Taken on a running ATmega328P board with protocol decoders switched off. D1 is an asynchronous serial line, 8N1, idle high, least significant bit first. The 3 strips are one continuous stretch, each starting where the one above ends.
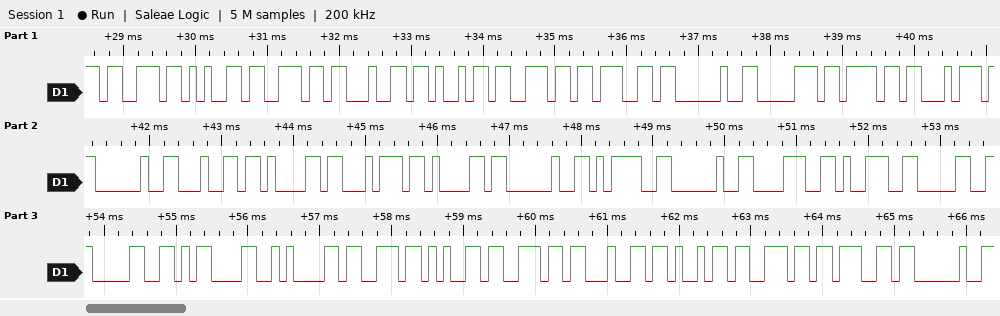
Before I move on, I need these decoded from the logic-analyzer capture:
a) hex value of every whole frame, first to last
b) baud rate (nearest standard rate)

73 65 6E 64 69 6E 67 20 70 6F 74 20 64 61 74 61 20 3D 20 38 39 30 30 0D 0A 73 65 6E 64 69 6E 67 20
9600 baud
